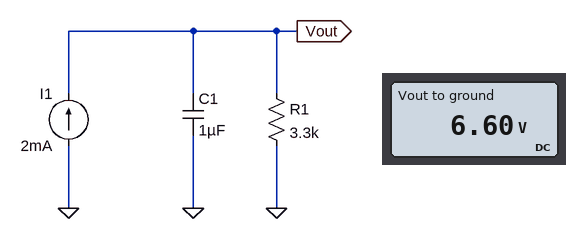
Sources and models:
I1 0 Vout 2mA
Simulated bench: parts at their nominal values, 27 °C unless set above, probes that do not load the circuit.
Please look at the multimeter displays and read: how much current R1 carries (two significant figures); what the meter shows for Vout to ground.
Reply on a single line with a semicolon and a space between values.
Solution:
2.0 mA; 6.60 V
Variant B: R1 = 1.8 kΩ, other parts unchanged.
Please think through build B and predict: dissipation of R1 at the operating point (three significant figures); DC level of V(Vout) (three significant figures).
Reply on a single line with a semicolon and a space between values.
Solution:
7.20 mW; 3.60 V
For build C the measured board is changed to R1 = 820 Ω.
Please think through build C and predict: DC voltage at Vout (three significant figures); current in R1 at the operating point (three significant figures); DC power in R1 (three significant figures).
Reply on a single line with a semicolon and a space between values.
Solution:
1.64 V; 2.00 mA; 3.28 mW
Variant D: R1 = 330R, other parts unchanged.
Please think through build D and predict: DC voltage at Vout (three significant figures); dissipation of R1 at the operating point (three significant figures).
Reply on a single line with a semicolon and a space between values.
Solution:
660 mV; 1.32 mW
